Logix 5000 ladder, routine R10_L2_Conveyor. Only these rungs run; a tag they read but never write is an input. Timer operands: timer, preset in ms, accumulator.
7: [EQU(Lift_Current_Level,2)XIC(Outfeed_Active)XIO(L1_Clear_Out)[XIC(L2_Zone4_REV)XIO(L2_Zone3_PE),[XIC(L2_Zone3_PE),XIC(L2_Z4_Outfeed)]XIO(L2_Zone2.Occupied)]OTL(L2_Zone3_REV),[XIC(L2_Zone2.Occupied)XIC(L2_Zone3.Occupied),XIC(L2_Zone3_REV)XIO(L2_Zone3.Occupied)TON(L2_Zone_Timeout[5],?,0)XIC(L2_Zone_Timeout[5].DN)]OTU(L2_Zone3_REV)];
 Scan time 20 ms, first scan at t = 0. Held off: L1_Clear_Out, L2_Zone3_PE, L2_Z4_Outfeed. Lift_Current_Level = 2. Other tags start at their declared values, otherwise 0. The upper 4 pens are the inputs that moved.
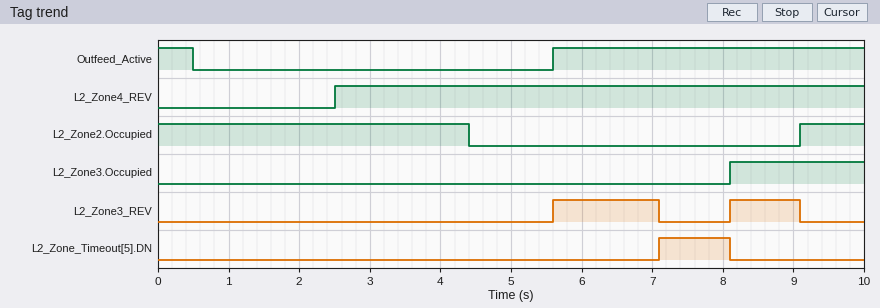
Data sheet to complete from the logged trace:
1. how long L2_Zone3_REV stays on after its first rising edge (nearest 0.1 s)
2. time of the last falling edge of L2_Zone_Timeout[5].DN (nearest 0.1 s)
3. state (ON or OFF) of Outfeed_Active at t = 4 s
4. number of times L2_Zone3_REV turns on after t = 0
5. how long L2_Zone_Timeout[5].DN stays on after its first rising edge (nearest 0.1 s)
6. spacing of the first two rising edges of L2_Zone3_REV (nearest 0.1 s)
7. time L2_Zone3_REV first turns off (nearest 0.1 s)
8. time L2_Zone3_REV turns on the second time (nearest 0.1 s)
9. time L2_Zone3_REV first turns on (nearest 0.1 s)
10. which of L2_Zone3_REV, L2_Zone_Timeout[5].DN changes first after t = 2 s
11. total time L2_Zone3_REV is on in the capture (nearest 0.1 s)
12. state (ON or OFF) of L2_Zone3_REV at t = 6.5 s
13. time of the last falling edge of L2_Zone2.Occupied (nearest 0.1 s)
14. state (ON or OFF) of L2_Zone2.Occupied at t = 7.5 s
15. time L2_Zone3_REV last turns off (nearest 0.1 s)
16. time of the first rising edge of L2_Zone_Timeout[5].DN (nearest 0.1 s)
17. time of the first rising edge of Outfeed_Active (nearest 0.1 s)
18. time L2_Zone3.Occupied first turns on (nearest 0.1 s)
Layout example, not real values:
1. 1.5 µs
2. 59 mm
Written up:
1. 1.5 s
2. 8.1 s
3. OFF
4. 2
5. 1.0 s
6. 2.5 s
7. 7.1 s
8. 8.1 s
9. 5.6 s
10. L2_Zone3_REV
11. 2.5 s
12. ON
13. 4.4 s
14. OFF
15. 9.1 s
16. 7.1 s
17. 5.6 s
18. 8.1 s
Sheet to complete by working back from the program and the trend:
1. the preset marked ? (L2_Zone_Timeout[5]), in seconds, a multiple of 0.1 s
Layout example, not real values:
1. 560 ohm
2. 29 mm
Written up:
1. 1.5 s
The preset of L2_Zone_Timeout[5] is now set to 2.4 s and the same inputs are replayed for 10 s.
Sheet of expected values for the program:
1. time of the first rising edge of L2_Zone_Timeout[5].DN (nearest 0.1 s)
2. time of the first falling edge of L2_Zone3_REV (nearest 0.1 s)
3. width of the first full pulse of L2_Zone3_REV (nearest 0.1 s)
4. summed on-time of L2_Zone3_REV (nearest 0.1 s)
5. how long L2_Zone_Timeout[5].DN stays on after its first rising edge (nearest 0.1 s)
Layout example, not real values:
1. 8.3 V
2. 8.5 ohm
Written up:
1. 8.0 s
2. 8.0 s
3. 2.4 s
4. 3.4 s
5. 0.1 s
